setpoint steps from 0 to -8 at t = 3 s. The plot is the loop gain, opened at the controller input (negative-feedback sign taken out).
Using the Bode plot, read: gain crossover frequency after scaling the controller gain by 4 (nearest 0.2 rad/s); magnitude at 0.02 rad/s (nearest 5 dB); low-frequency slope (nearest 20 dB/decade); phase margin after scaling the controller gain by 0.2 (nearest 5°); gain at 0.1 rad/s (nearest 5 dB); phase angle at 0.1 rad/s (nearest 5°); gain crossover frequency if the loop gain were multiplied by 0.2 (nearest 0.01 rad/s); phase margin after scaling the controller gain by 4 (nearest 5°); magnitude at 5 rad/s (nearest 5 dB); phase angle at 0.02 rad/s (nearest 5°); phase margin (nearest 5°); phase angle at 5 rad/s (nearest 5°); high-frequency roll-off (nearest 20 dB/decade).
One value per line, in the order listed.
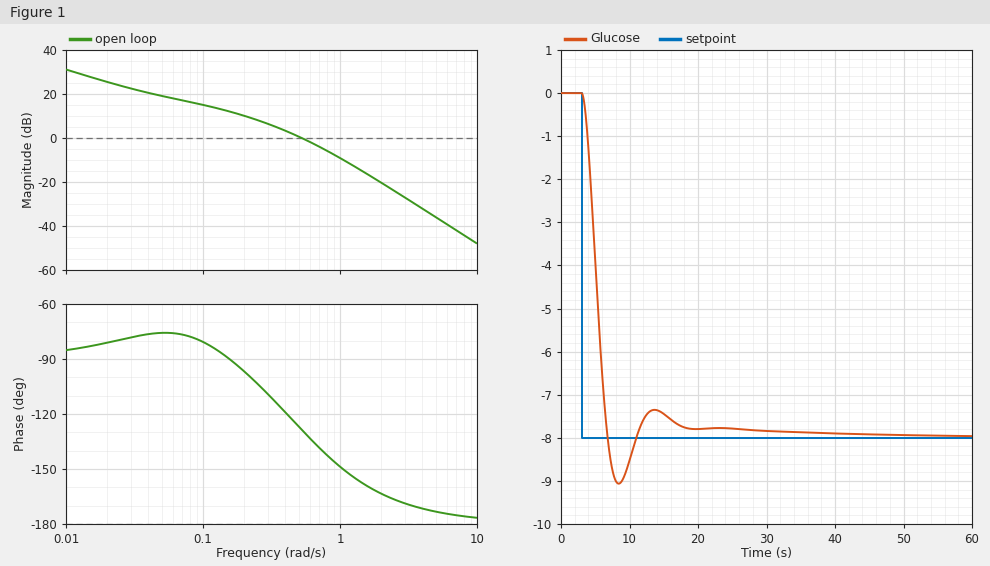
1.2 rad/s
25 dB
-20 dB/decade
95°
15 dB
-80°
0.12 rad/s
25°
-35 dB
-80°
50°
-175°
-40 dB/decade
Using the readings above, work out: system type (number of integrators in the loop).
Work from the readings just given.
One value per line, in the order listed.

1
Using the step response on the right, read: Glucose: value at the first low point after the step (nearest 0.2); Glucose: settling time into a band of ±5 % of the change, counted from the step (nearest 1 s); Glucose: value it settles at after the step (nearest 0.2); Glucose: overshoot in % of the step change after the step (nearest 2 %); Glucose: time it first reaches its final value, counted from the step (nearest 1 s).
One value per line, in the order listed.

-9.0
13 s
-8.0
14 %
4 s
